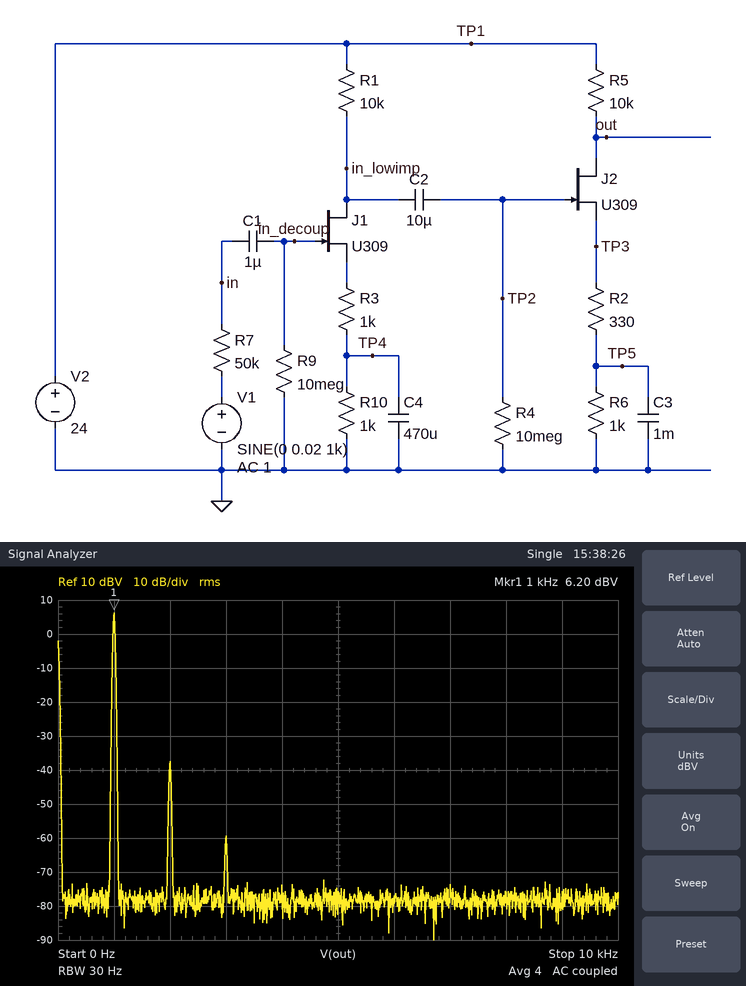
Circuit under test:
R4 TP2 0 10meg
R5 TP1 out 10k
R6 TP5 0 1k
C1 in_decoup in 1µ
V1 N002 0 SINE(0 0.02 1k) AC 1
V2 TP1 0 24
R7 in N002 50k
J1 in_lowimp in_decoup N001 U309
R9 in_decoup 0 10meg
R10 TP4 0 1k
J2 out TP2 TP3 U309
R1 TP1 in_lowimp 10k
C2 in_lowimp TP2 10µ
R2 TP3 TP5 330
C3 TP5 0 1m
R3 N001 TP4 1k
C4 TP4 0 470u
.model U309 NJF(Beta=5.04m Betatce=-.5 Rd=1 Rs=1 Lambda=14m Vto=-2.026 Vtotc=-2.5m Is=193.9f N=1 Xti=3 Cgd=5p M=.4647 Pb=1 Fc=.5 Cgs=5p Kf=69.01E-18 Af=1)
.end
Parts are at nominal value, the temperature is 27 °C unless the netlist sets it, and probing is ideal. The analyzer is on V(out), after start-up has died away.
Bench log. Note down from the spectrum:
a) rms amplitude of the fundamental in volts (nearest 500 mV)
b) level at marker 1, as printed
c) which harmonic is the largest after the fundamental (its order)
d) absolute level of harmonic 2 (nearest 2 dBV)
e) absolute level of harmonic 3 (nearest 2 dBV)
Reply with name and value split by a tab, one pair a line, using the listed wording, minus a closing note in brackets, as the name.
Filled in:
rms amplitude of the fundamental in volts	2.0 V
level at marker 1, as printed	6.20 dBV
which harmonic is the largest after the fundamental	2
absolute level of harmonic 2	-38 dBV
absolute level of harmonic 3	-60 dBV
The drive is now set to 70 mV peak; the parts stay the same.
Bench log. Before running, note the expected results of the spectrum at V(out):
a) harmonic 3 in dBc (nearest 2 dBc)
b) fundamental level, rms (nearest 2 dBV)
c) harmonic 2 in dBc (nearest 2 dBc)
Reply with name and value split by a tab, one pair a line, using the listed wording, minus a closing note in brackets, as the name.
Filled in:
harmonic 3 in dBc	-36 dBc
fundamental level, rms	16 dBV
harmonic 2 in dBc	-34 dBc
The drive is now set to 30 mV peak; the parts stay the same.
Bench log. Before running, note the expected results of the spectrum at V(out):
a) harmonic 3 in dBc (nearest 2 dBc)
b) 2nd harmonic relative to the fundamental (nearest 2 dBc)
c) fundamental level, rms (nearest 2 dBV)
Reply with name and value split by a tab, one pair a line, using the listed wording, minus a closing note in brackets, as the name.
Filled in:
harmonic 3 in dBc	-58 dBc
2nd harmonic relative to the fundamental	-40 dBc
fundamental level, rms	10 dBV
